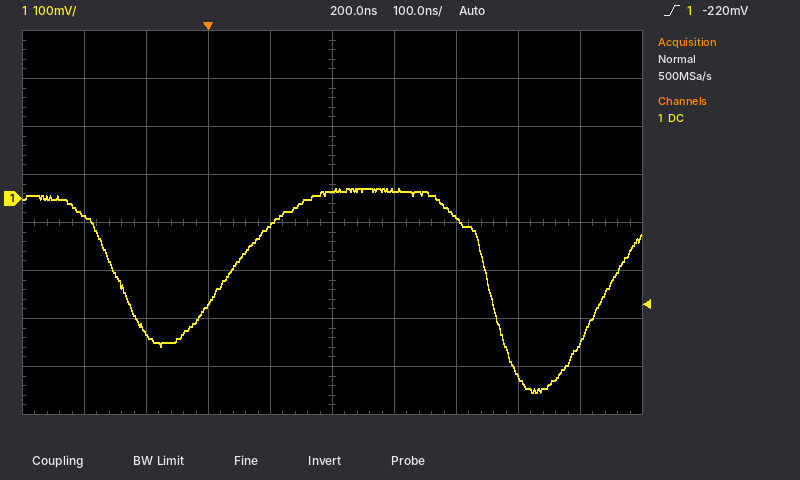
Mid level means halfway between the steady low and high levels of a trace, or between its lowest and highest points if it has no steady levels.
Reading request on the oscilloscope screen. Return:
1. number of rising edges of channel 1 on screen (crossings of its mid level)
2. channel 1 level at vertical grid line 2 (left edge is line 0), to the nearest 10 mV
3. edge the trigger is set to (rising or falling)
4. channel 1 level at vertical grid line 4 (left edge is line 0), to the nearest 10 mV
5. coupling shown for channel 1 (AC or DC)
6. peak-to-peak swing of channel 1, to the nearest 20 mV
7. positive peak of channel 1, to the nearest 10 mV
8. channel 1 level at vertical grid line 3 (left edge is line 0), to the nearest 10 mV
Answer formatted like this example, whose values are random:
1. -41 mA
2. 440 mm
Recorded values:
1. 2
2. -280 mV
3. rising
4. -60 mV
5. DC
6. 420 mV
7. 20 mV
8. -220 mV
